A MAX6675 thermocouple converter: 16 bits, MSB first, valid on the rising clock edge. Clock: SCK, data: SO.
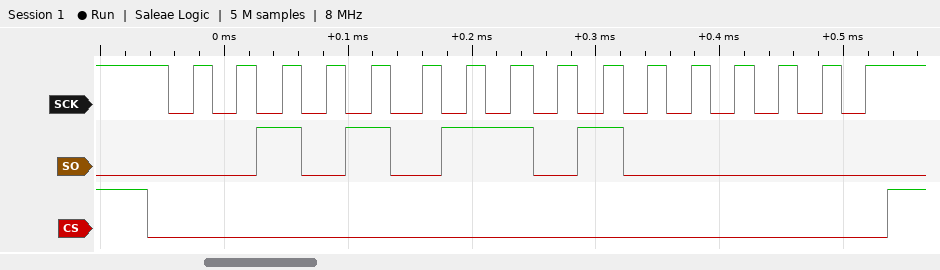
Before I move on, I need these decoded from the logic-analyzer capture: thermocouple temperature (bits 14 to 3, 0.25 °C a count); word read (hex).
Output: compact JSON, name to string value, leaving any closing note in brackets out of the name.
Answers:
{"thermocouple temperature": "346.00 °C", "word read": "0x2B40"}
